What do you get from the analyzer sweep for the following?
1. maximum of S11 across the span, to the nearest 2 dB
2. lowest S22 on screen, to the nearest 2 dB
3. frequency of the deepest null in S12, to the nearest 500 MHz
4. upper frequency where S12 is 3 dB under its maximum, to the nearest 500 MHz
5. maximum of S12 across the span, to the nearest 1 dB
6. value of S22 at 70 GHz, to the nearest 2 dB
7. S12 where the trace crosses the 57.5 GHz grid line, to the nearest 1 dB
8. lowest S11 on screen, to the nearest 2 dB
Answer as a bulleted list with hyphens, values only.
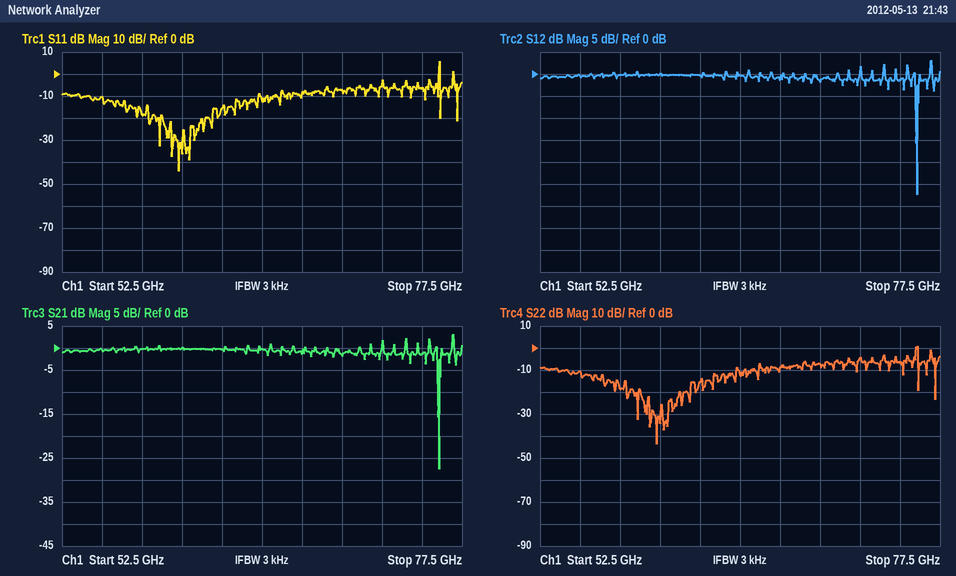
- 6 dB
- -44 dB
- 76.0 GHz
- 77.0 GHz
- 3 dB
- -8 dB
- 0 dB
- -44 dB
